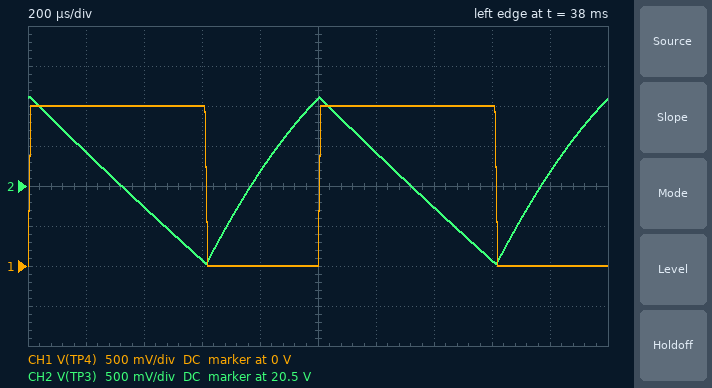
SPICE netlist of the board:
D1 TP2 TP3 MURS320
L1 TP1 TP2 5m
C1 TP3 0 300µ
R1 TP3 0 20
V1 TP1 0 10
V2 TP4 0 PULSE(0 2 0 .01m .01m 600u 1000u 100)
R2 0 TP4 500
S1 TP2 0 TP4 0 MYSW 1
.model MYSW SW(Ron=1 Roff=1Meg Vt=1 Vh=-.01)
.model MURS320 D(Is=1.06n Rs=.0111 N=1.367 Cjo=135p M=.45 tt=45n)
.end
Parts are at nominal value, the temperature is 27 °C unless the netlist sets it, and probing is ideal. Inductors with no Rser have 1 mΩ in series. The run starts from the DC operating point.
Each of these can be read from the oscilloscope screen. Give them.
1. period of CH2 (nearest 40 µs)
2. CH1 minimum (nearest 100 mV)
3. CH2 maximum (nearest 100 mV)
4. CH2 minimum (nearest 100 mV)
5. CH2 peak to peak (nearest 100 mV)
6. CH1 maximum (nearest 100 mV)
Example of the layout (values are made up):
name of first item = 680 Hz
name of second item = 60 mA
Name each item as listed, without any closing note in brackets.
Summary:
period of CH2 = 1.00 ms
CH1 minimum = 0 V
CH2 maximum = 21.6 V
CH2 minimum = 19.5 V
CH2 peak to peak = 2.1 V
CH1 maximum = 2.0 V
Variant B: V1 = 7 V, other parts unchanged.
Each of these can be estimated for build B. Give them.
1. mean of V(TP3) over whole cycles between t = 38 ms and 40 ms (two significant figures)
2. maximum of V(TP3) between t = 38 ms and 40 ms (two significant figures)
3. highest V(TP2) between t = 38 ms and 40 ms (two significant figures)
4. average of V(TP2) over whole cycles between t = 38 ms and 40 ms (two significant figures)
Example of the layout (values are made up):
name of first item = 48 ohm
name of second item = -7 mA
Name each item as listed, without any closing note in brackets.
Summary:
mean of V(TP3) over whole cycles between t = 38 ms and 40 ms = 14 V
maximum of V(TP3) between t = 38 ms and 40 ms = 15 V
highest V(TP2) between t = 38 ms and 40 ms = 16 V
average of V(TP2) over whole cycles between t = 38 ms and 40 ms = 7.0 V
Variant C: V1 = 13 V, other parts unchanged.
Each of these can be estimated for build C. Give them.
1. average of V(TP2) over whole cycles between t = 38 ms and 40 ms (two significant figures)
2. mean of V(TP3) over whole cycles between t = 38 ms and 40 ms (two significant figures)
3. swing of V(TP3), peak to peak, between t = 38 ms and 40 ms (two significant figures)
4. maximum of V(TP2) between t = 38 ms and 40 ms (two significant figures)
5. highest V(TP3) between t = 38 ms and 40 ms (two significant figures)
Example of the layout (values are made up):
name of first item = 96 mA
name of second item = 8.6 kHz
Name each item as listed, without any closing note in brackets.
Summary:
average of V(TP2) over whole cycles between t = 38 ms and 40 ms = 13 V
mean of V(TP3) over whole cycles between t = 38 ms and 40 ms = 27 V
swing of V(TP3), peak to peak, between t = 38 ms and 40 ms = 2.7 V
maximum of V(TP2) between t = 38 ms and 40 ms = 29 V
highest V(TP3) between t = 38 ms and 40 ms = 28 V
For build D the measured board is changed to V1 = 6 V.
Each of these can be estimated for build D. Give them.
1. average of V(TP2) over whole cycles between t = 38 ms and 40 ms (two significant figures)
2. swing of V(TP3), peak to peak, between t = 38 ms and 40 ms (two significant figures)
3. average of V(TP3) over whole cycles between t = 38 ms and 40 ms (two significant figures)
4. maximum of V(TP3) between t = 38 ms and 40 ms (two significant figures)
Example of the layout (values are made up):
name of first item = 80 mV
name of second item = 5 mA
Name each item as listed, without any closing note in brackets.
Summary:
average of V(TP2) over whole cycles between t = 38 ms and 40 ms = 6.0 V
swing of V(TP3), peak to peak, between t = 38 ms and 40 ms = 1.2 V
average of V(TP3) over whole cycles between t = 38 ms and 40 ms = 12 V
maximum of V(TP3) between t = 38 ms and 40 ms = 13 V
